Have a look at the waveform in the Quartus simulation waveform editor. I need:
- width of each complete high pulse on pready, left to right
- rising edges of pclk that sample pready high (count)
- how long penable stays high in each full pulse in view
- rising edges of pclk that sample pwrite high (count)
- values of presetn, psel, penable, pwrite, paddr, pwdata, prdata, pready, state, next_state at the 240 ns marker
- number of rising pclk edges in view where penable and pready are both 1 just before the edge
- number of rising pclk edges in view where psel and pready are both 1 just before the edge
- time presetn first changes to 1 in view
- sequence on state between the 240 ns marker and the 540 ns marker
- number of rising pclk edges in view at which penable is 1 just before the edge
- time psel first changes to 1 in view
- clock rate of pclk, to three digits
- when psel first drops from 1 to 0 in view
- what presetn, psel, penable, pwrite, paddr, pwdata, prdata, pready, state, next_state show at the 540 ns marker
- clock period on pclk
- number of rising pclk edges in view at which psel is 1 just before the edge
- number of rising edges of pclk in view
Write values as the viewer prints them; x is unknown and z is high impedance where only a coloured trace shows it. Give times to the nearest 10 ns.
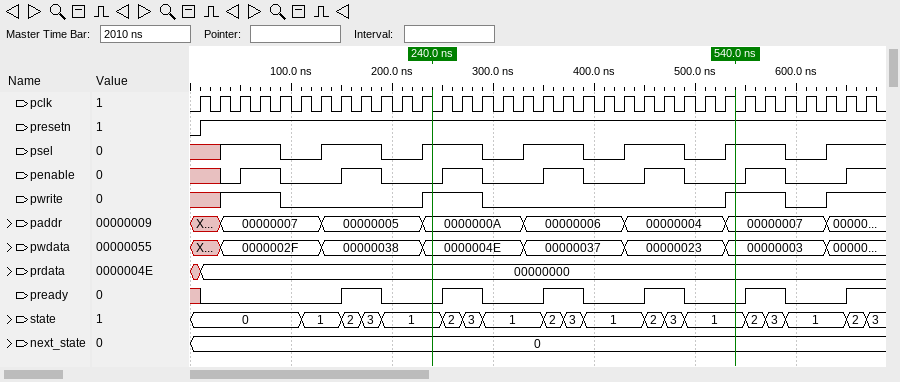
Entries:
40 ns, 40 ns, 40 ns, 40 ns, 40 ns
11
40 ns, 40 ns, 40 ns, 40 ns, 40 ns, 40 ns
11
presetn=1, psel=1, penable=0, pwrite=1, paddr=0000000A, pwdata=0000004E, prdata=00000000, pready=0, state=1, next_state=0
11
11
10 ns
1, 2, 3, 1, 2, 3, 1, 2, 3, 1
13
30 ns
50.0 MHz
90 ns
presetn=1, psel=1, penable=0, pwrite=1, paddr=00000007, pwdata=00000003, prdata=00000000, pready=0, state=1, next_state=0
20 ns
20
34
